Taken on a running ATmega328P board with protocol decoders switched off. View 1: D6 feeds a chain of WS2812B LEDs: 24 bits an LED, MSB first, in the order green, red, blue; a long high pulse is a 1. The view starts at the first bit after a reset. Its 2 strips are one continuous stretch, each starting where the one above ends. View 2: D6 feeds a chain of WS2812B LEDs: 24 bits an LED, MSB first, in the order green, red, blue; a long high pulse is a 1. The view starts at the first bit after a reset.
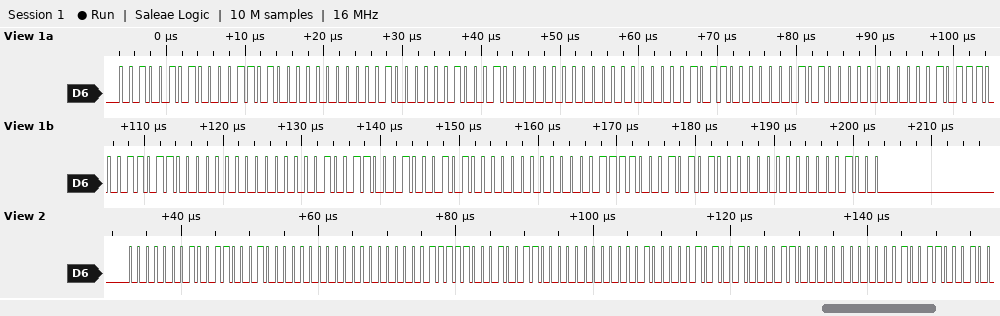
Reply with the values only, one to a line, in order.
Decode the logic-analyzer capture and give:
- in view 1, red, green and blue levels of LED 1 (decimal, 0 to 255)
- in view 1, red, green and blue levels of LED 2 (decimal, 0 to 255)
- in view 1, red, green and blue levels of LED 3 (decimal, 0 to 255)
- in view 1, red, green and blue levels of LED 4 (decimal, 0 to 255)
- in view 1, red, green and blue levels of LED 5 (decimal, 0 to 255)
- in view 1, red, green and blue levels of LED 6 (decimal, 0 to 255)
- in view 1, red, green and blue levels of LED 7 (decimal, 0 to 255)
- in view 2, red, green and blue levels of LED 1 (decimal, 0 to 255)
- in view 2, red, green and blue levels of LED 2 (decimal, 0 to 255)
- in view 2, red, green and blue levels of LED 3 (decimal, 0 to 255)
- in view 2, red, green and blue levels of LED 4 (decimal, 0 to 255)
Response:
13, 37, 0
34, 16, 0
44, 0, 5
23, 0, 27
1, 0, 49
0, 20, 30
0, 42, 8
49, 1, 0
31, 0, 19
8, 0, 41
0, 12, 38
